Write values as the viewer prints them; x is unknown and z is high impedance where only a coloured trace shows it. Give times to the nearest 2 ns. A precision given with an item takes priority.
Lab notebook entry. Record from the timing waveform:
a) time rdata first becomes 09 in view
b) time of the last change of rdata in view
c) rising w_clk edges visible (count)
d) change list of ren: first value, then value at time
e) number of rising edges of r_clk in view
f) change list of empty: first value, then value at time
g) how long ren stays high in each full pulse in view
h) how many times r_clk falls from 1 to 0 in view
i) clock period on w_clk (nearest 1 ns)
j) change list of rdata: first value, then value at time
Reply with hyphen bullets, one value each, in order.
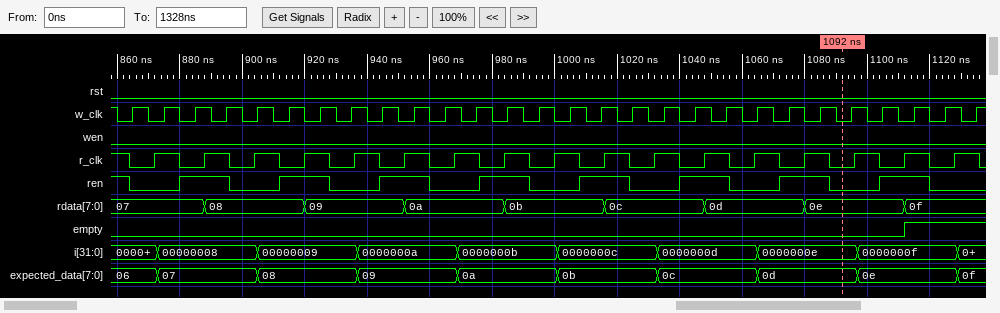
- 920 ns
- 1112 ns
- 28
- 1, 0 at 864 ns, 1 at 880 ns, 0 at 896 ns, 1 at 912 ns, 0 at 928 ns, 1 at 944 ns, 0 at 960 ns, 1 at 976 ns, 0 at 992 ns, 1 at 1008 ns, 0 at 1024 ns, 1 at 1040 ns, 0 at 1056 ns, 1 at 1072 ns, 0 at 1088 ns, 1 at 1104 ns, 0 at 1120 ns
- 17
- 0, 1 at 1112 ns
- 16 ns, 16 ns, 16 ns, 16 ns, 16 ns, 16 ns, 16 ns, 16 ns
- 18
- 10 ns
- 07, 08 at 888 ns, 09 at 920 ns, 0a at 952 ns, 0b at 984 ns, 0c at 1016 ns, 0d at 1048 ns, 0e at 1080 ns, 0f at 1112 ns
